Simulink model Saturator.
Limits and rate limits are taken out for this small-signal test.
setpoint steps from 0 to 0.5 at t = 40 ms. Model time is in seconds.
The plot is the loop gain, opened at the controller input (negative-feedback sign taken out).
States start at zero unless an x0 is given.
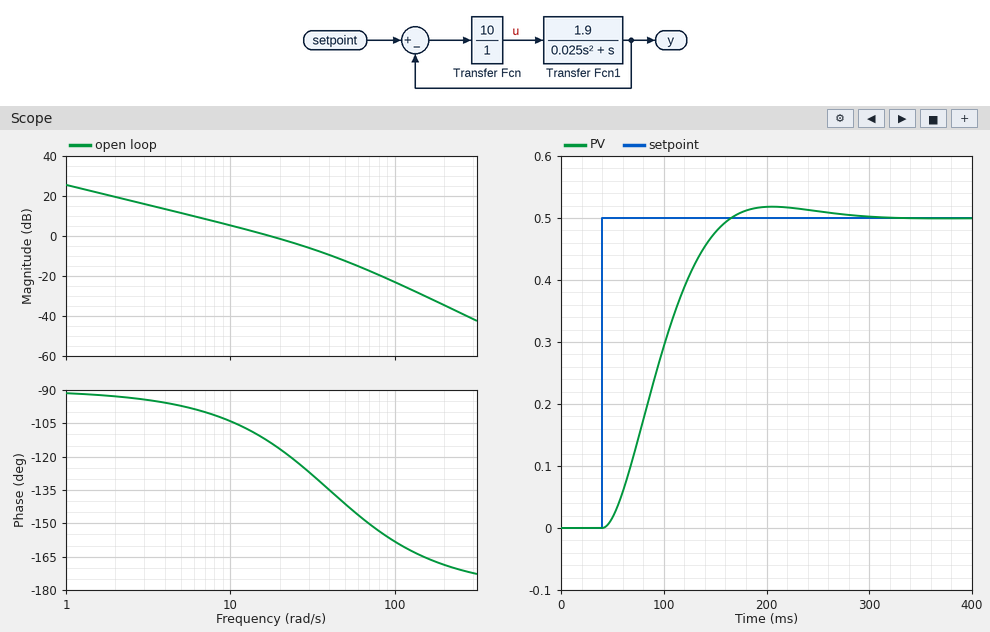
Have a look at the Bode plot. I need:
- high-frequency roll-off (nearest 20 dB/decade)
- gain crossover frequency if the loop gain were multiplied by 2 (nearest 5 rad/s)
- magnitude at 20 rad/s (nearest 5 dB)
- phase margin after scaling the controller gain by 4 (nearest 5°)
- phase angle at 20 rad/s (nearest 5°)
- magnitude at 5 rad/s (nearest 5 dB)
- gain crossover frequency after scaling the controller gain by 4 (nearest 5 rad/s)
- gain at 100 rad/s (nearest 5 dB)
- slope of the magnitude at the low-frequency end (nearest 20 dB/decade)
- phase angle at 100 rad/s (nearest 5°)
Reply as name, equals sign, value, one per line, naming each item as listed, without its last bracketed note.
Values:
high-frequency roll-off = -40 dB/decade
gain crossover frequency if the loop gain were multiplied by 2 = 30 rad/s
magnitude at 20 rad/s = 0 dB
phase margin after scaling the controller gain by 4 = 40°
phase angle at 20 rad/s = -115°
magnitude at 5 rad/s = 10 dB
gain crossover frequency after scaling the controller gain by 4 = 50 rad/s
gain at 100 rad/s = -25 dB
slope of the magnitude at the low-frequency end = -20 dB/decade
phase angle at 100 rad/s = -160°
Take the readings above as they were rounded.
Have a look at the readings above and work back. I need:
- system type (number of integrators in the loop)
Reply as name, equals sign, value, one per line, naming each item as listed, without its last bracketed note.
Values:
system type = 1
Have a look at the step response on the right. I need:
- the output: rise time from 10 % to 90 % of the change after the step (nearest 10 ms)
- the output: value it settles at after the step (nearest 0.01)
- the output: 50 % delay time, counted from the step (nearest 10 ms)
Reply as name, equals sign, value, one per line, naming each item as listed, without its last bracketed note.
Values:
the output: rise time from 10 % to 90 % of the change after the step = 80 ms
the output: value it settles at after the step = 0.50
the output: 50 % delay time, counted from the step = 50 ms
